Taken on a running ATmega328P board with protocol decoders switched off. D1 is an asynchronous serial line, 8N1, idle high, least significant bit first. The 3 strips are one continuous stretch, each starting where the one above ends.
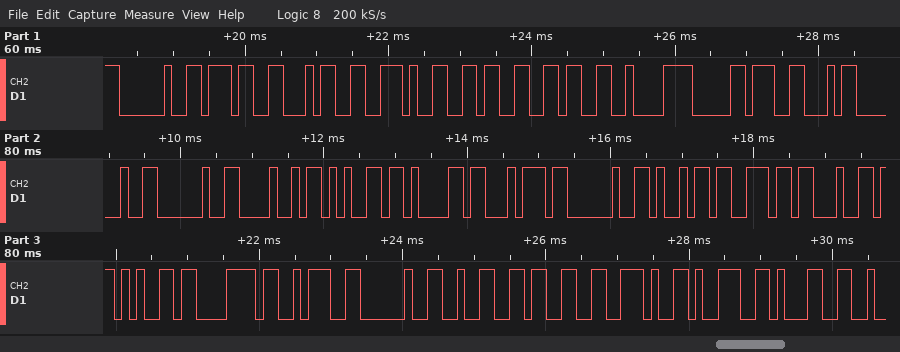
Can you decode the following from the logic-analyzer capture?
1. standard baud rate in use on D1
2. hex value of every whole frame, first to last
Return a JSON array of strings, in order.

["9600 baud", "20 37 34 2E 36 36 C2 B0 46 20 20 48 65 61 74 20 69 6E 64 65 78 3A 20 32 33 2E 39 31"]
